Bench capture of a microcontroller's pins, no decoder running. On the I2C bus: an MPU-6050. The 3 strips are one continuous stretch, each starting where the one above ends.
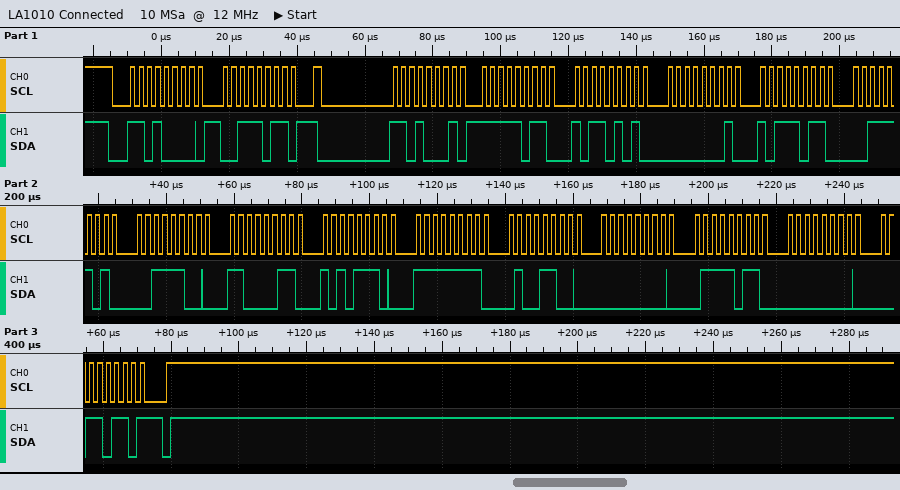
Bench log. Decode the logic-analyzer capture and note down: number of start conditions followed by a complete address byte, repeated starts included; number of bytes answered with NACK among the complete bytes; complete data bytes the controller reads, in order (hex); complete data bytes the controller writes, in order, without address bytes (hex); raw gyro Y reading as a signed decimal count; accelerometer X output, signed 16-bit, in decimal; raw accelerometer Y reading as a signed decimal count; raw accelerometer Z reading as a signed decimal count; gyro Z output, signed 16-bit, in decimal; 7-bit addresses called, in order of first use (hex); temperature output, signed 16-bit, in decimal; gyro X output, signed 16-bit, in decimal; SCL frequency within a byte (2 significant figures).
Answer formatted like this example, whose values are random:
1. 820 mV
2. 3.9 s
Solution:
1. 2
2. 1
3. FB B5 01 BB 3D 3C C3 AE FF 4C 00 7B 00 36
4. 3B
5. 123
6. -1099
7. 443
8. 15676
9. 54
10. 0x68
11. -15442
12. -180
13. 400 kHz
